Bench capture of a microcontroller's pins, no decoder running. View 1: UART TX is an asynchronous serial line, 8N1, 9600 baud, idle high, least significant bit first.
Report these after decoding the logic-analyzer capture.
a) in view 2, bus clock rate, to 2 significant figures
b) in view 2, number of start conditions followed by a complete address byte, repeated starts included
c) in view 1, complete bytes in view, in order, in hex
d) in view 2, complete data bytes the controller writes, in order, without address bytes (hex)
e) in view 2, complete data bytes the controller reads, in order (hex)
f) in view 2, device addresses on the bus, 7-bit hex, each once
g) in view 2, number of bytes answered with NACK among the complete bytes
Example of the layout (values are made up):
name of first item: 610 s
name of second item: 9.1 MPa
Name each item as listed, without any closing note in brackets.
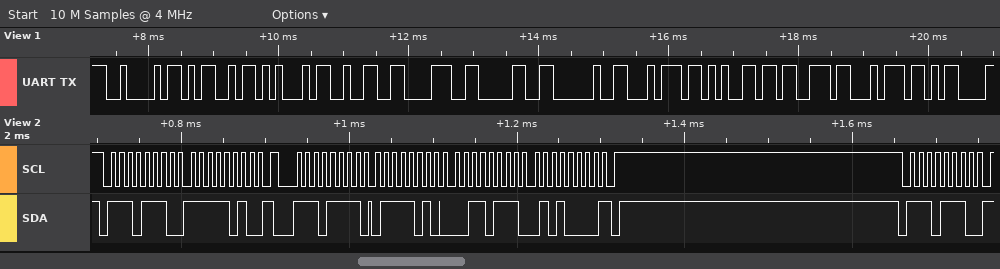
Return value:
in view 2, bus clock rate, to 2 significant figures: 100 kHz
in view 2, number of start conditions followed by a complete address byte, repeated starts included: 3
in view 1, complete bytes in view, in order, in hex: 42 4D 45 32 38 30 20 74 65 73 74 0D
in view 2, complete data bytes the controller writes, in order, without address bytes: FA
in view 2, complete data bytes the controller reads, in order: 7A 37 50
in view 2, device addresses on the bus, 7-bit hex, each once: 0x77
in view 2, number of bytes answered with NACK among the complete bytes: 1
